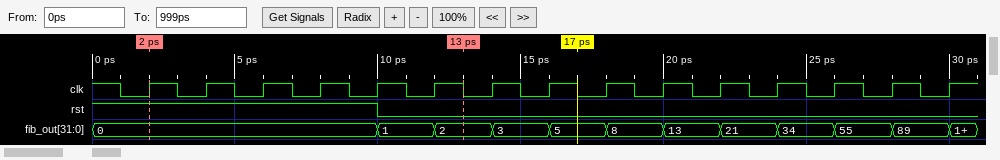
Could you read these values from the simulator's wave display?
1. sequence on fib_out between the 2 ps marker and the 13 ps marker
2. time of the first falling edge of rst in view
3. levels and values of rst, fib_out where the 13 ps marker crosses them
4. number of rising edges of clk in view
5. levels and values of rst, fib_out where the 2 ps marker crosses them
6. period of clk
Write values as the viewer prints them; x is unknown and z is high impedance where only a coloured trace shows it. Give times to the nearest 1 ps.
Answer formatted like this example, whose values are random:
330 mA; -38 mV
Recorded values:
0, 1, 2; 10 ps; rst=0, fib_out=2; 15; rst=1, fib_out=0; 2 ps
